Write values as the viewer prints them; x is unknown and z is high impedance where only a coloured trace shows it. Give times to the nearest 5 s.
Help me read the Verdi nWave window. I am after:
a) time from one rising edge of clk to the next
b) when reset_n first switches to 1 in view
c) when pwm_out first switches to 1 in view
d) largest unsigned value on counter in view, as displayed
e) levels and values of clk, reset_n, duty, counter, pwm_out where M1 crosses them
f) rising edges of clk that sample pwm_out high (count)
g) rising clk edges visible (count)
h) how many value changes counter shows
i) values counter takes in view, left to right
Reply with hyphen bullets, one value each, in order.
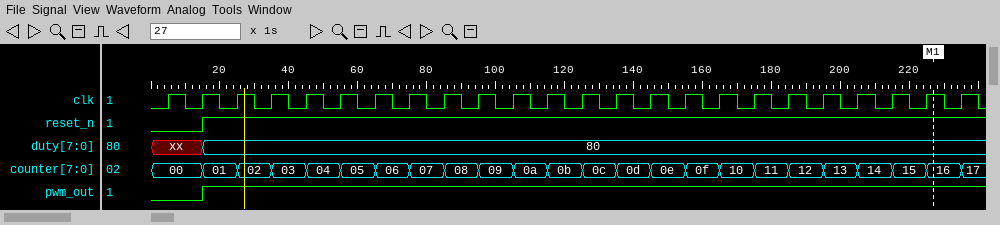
- 10 s
- 15 s
- 15 s
- 17
- clk=1, reset_n=1, duty=80, counter=16, pwm_out=1
- 22
- 24
- 23
- 00, 01, 02, 03, 04, 05, 06, 07, 08, 09, 0a, 0b, 0c, 0d, 0e, 0f, 10, 11, 12, 13, 14, 15, 16, 17
